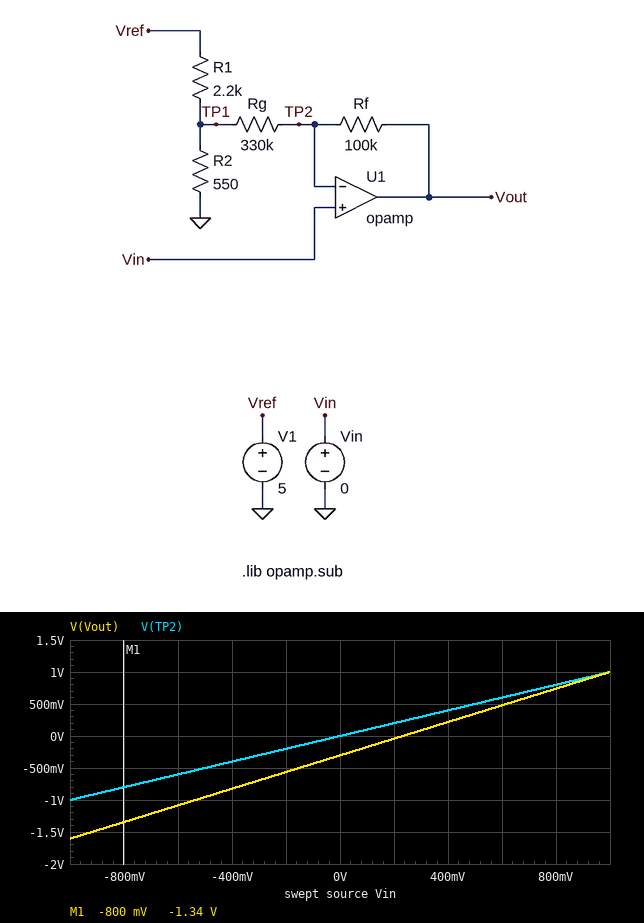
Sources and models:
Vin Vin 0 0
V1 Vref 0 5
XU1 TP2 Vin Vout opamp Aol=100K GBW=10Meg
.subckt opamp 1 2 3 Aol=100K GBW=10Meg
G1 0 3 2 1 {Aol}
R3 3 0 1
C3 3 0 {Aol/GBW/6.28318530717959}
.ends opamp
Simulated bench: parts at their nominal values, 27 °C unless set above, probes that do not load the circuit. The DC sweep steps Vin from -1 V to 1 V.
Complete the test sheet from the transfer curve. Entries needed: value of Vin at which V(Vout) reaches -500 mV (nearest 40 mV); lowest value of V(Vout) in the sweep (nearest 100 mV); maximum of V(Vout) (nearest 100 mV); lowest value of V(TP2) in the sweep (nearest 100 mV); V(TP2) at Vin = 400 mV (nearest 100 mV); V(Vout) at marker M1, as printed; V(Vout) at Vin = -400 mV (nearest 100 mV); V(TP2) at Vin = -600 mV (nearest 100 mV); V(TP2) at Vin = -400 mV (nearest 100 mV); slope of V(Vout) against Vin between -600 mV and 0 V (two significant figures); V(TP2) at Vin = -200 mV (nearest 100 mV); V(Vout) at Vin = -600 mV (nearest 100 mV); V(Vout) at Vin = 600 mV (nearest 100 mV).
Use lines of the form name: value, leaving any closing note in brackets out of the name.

value of Vin at which V(Vout) reaches -500 mV: -160 mV
lowest value of V(Vout) in the sweep: -1.6 V
maximum of V(Vout): 1.0 V
lowest value of V(TP2) in the sweep: -1.0 V
V(TP2) at Vin = 400 mV: 400 mV
V(Vout) at marker M1, as printed: -1.34 V
V(Vout) at Vin = -400 mV: -800 mV
V(TP2) at Vin = -600 mV: -600 mV
V(TP2) at Vin = -400 mV: -400 mV
slope of V(Vout) against Vin between -600 mV and 0 V: 1.3 V/V
V(TP2) at Vin = -200 mV: -200 mV
V(Vout) at Vin = -600 mV: -1.1 V
V(Vout) at Vin = 600 mV: 500 mV
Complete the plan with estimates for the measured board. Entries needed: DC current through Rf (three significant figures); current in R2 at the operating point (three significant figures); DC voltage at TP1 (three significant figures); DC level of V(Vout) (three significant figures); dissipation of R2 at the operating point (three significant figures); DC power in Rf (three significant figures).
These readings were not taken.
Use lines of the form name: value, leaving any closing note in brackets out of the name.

DC current through Rf: 3.03 µA
current in R2 at the operating point: 1.82 mA
DC voltage at TP1: 999 mV
DC level of V(Vout): -303 mV
dissipation of R2 at the operating point: 1.81 mW
DC power in Rf: 916 nW
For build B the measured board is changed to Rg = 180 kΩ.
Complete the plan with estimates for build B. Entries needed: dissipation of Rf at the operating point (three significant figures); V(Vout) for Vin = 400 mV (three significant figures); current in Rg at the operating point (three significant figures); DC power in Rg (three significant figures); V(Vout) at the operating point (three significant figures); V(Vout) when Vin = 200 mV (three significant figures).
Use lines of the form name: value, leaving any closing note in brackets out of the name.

dissipation of Rf at the operating point: 3.07 µW
V(Vout) for Vin = 400 mV: 67.5 mV
current in Rg at the operating point: 5.54 µA
DC power in Rg: 5.53 µW
V(Vout) at the operating point: -554 mV
V(Vout) when Vin = 200 mV: -243 mV
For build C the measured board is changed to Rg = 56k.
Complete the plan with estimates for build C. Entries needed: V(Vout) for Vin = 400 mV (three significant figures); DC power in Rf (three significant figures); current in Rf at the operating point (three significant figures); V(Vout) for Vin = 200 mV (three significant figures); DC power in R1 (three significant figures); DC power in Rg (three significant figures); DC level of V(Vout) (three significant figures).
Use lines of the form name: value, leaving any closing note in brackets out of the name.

V(Vout) for Vin = 400 mV: -663 mV
DC power in Rf: 31.4 µW
current in Rf at the operating point: 17.7 µA
V(Vout) for Vin = 200 mV: -1.22 V
DC power in R1: 7.30 mW
DC power in Rg: 17.6 µW
DC level of V(Vout): -1.77 V
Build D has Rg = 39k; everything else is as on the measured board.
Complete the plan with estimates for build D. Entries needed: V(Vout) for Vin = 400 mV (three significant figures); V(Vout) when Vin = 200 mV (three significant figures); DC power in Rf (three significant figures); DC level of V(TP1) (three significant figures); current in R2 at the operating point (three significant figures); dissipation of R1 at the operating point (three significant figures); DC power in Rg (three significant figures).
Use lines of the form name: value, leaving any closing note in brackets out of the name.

V(Vout) for Vin = 400 mV: -1.12 V
V(Vout) when Vin = 200 mV: -1.83 V
DC power in Rf: 64.3 µW
DC level of V(TP1): 989 mV
current in R2 at the operating point: 1.80 mA
dissipation of R1 at the operating point: 7.31 mW
DC power in Rg: 25.1 µW
